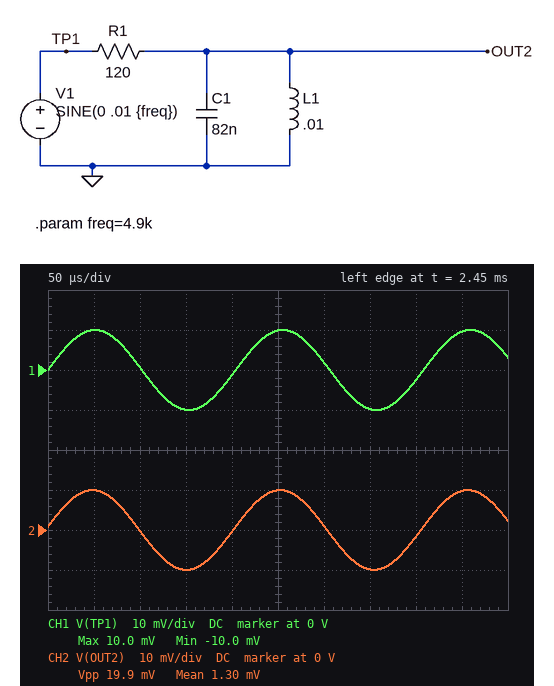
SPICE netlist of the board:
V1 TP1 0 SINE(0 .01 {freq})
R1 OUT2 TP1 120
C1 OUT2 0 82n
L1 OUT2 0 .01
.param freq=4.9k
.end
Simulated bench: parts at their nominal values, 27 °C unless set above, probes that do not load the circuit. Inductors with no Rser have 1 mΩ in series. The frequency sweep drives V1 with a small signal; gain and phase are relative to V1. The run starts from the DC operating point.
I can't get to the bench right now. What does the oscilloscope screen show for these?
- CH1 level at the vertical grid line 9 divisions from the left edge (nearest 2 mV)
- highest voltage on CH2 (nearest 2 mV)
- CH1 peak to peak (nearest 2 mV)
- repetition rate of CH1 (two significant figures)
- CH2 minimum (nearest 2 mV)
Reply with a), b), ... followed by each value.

a) 10 mV
b) 10 mV
c) 20 mV
d) 4.9 kHz
e) -10 mV
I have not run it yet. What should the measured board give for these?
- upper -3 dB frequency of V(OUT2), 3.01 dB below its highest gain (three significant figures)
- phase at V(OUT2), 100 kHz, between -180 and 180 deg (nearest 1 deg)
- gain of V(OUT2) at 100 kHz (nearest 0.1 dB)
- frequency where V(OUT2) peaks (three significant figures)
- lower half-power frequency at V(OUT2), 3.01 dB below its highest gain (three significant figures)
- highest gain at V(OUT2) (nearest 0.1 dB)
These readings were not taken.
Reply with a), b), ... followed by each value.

a) 17.9 kHz
b) -81 deg
c) -15.9 dB
d) 5.56 kHz
e) 1.73 kHz
f) 0 dB
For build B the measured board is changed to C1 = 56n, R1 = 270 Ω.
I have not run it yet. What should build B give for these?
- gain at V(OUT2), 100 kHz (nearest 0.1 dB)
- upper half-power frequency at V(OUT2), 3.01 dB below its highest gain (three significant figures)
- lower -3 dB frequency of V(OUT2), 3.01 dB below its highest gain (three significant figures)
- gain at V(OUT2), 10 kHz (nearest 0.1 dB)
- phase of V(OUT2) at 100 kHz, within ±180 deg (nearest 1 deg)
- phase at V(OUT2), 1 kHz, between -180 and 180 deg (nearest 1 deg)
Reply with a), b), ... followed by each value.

a) -19.6 dB
b) 13.8 kHz
c) 3.28 kHz
d) -1.0 dB
e) -84 deg
f) 77 deg
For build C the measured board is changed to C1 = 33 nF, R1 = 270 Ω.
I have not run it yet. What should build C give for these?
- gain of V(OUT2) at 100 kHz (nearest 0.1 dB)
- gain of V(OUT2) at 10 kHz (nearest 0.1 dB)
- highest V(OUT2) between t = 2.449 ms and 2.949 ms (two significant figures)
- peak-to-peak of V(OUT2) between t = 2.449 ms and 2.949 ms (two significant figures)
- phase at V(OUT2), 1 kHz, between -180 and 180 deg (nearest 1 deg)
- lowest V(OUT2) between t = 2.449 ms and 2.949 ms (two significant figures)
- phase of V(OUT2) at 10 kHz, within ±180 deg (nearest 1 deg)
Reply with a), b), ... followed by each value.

a) -15.0 dB
b) -0.1 dB
c) 8.6 mV
d) 17 mV
e) 77 deg
f) -8.6 mV
g) -7 deg
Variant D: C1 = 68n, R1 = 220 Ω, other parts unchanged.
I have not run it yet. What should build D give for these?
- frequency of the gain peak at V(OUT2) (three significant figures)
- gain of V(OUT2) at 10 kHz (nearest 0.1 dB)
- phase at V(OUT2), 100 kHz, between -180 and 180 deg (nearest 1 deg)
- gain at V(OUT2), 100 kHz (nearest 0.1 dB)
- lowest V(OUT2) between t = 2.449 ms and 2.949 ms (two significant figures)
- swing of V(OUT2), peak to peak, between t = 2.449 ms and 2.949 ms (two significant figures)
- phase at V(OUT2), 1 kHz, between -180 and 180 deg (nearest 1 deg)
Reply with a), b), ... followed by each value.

a) 6.10 kHz
b) -1.3 dB
c) -84 deg
d) -19.5 dB
e) -9.7 mV
f) 19 mV
g) 74 deg
